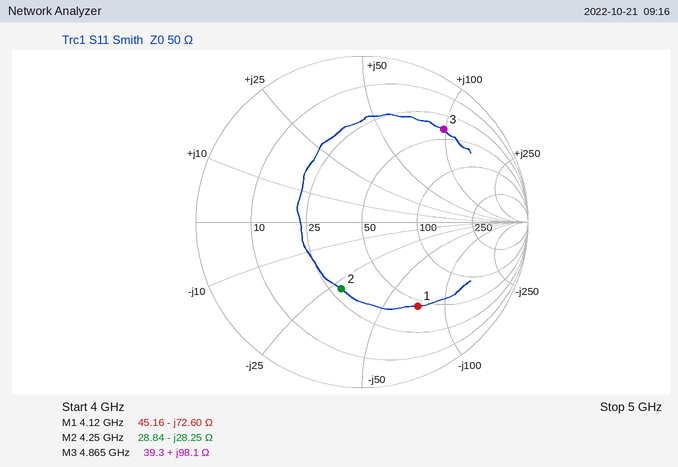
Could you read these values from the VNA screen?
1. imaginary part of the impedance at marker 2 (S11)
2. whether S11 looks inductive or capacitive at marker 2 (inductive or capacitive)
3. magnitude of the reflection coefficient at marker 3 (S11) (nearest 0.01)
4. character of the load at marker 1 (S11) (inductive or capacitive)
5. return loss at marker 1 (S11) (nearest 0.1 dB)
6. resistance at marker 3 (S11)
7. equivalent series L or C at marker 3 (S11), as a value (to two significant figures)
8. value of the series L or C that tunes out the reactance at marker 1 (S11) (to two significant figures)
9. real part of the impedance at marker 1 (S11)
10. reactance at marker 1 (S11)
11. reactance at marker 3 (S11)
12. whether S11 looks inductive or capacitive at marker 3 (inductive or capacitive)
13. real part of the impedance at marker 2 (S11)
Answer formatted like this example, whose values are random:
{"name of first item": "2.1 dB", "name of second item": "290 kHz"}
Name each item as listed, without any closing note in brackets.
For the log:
{"imaginary part of the impedance at marker 2": "-28.25 Ω", "whether S11 looks inductive or capacitive at marker 2": "capacitive", "magnitude of the reflection coefficient at marker 3 (S11)": "0.74", "character of the load at marker 1 (S11)": "capacitive", "return loss at marker 1 (S11)": "4.3 dB", "resistance at marker 3": "39.3 Ω", "equivalent series L or C at marker 3 (S11), as a value": "3.2 nH", "value of the series L or C that tunes out the reactance at marker 1 (S11)": "2.8 nH", "real part of the impedance at marker 1": "45.16 Ω", "reactance at marker 1": "-72.60 Ω", "reactance at marker 3": "+98.1 Ω", "whether S11 looks inductive or capacitive at marker 3": "inductive", "real part of the impedance at marker 2": "28.84 Ω"}
